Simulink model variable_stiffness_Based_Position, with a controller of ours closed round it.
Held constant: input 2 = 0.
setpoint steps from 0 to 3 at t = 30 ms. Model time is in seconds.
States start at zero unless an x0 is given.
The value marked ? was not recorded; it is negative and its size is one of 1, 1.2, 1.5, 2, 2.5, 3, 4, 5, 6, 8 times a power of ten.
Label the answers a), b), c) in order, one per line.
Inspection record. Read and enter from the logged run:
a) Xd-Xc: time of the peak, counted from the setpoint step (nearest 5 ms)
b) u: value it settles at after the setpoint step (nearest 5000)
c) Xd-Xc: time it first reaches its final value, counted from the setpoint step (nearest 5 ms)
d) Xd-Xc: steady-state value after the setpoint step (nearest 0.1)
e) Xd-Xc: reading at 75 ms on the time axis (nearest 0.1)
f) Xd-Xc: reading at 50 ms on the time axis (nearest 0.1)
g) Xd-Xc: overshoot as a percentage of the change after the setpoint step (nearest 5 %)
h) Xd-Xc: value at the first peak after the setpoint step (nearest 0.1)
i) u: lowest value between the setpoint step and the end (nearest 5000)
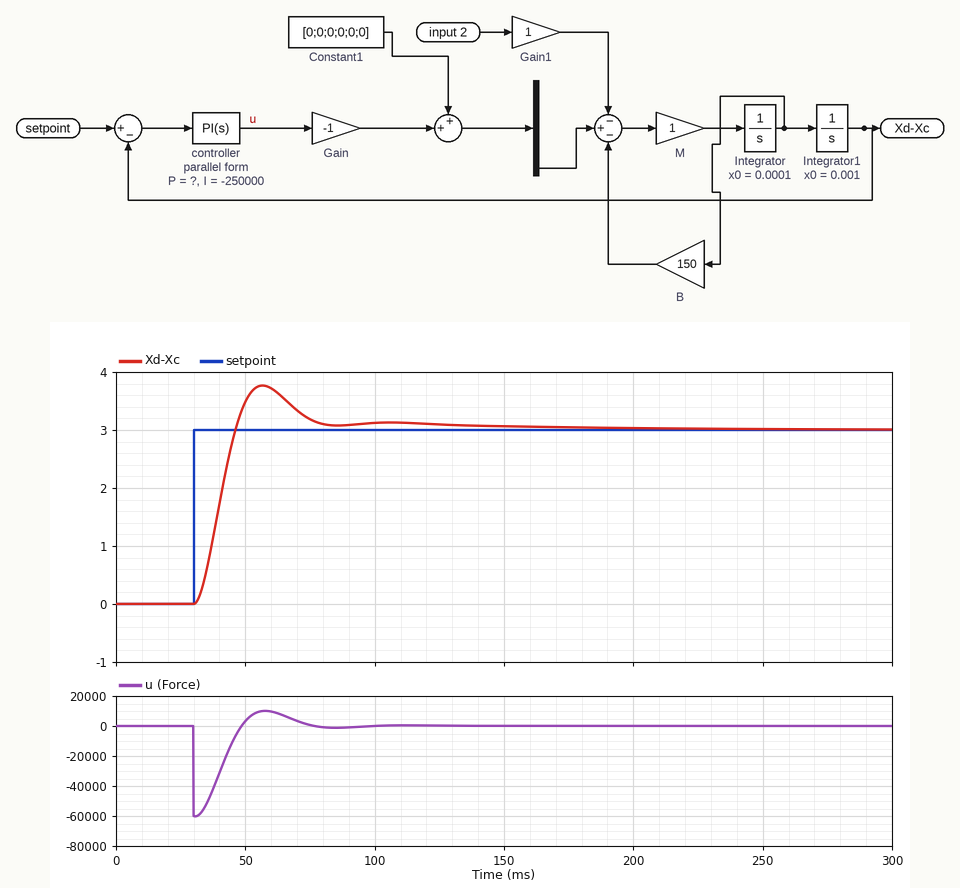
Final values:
a) 25 ms
b) 0
c) 15 ms
d) 3.0
e) 3.2
f) 3.5
g) 25 %
h) 3.8
i) -60000
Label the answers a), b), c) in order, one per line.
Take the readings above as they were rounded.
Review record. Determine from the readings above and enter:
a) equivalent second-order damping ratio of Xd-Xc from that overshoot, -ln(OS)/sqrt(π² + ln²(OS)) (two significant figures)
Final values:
a) 0.40
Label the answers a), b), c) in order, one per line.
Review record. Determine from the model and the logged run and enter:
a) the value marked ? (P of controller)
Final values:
a) -20000
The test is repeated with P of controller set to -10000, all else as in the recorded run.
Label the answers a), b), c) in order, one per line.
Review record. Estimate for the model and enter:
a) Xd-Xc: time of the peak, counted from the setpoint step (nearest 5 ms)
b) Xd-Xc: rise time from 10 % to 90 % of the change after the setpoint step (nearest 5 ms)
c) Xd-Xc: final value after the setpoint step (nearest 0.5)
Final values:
a) 45 ms
b) 15 ms
c) 3.0
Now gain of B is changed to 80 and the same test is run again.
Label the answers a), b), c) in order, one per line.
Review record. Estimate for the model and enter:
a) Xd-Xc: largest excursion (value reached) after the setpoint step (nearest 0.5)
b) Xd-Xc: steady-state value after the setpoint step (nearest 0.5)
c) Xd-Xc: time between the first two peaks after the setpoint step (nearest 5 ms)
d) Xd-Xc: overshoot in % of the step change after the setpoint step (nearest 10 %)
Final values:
a) 4.5
b) 3.0
c) 45 ms
d) 50 %
